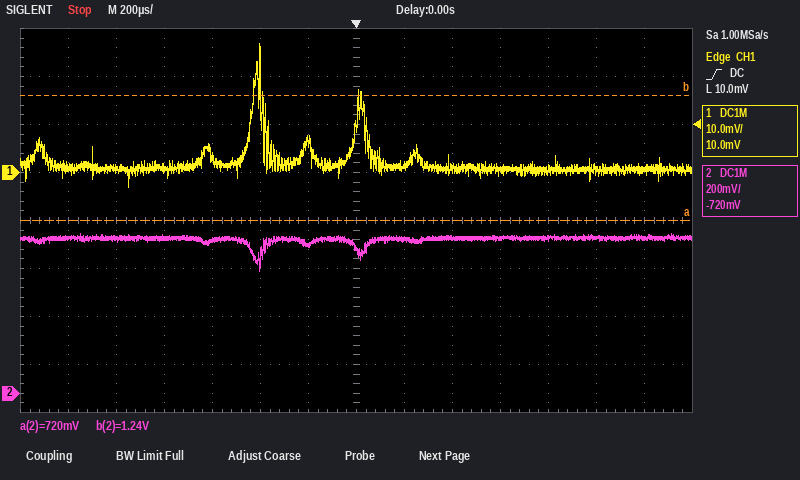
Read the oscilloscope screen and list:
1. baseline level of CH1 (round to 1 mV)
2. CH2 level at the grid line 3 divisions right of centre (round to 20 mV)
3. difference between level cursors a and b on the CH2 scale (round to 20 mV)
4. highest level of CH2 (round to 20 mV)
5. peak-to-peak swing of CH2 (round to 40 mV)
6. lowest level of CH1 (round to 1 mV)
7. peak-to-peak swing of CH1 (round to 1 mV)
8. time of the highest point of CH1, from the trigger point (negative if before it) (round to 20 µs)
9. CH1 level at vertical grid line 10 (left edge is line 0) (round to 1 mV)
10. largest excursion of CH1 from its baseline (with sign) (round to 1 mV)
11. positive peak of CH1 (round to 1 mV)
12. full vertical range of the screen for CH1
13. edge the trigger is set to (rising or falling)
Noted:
1 mV
640 mV
520 mV
660 mV
160 mV
-3 mV
30 mV
-400 µs
0 mV
+26 mV
27 mV
80 mV
rising
